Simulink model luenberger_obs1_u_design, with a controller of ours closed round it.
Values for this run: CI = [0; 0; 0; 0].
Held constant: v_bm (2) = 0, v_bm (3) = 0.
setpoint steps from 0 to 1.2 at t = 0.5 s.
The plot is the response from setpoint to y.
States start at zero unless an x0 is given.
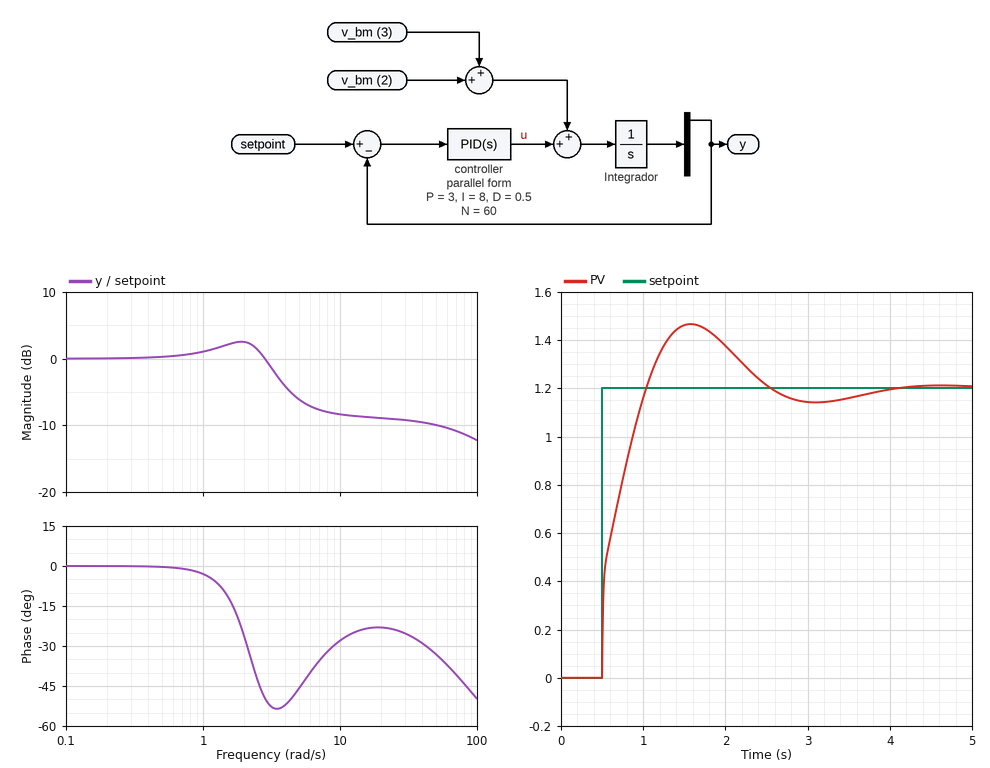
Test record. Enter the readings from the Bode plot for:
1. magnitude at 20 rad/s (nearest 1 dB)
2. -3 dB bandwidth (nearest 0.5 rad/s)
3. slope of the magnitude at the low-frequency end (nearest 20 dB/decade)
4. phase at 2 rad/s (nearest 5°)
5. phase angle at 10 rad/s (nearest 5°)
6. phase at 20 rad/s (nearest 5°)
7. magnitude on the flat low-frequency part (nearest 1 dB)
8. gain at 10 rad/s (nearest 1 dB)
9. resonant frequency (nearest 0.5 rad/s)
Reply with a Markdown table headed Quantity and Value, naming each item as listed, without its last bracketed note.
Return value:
| Quantity | Value |
|---|---|
| magnitude at 20 rad/s | -9 dB |
| -3 dB bandwidth | 3.5 rad/s |
| slope of the magnitude at the low-frequency end | 0 dB/decade |
| phase at 2 rad/s | -25° |
| phase angle at 10 rad/s | -30° |
| phase at 20 rad/s | -25° |
| magnitude on the flat low-frequency part | 0 dB |
| gain at 10 rad/s | -8 dB |
| resonant frequency | 2.0 rad/s |
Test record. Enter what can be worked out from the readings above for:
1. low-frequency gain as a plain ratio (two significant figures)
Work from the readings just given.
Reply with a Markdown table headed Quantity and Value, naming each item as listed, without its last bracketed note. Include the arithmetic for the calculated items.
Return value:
| Quantity | Value |
|---|---|
| low-frequency gain as a plain ratio | 10^(0 / 20) = 1.0 |
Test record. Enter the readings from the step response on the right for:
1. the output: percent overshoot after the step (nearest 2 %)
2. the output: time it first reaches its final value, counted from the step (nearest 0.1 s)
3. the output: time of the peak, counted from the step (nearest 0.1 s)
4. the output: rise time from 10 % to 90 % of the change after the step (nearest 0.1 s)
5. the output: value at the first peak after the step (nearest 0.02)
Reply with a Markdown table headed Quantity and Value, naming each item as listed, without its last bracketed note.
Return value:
| Quantity | Value |
|---|---|
| the output: percent overshoot after the step | 22 % |
| the output: time it first reaches its final value, counted from the step | 0.5 s |
| the output: time of the peak, counted from the step | 1.1 s |
| the output: rise time from 10 % to 90 % of the change after the step | 0.4 s |
| the output: value at the first peak after the step | 1.46 |
